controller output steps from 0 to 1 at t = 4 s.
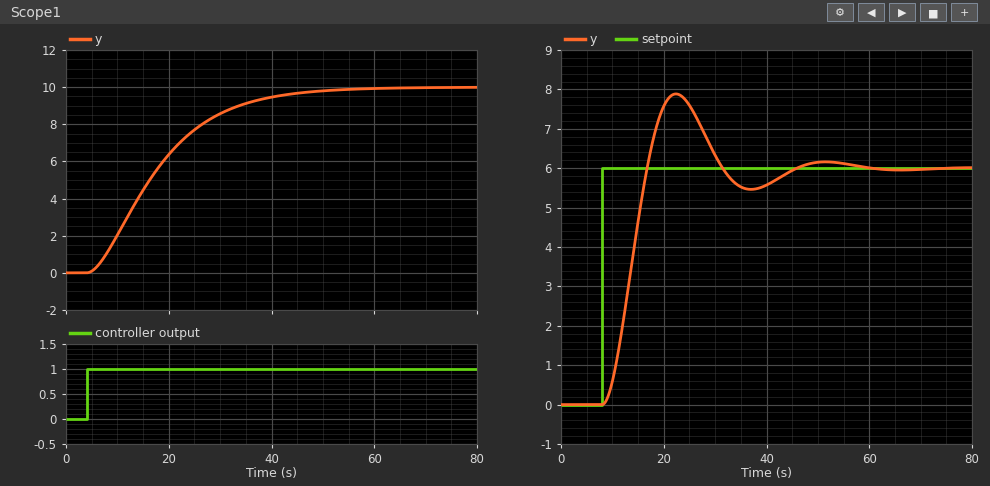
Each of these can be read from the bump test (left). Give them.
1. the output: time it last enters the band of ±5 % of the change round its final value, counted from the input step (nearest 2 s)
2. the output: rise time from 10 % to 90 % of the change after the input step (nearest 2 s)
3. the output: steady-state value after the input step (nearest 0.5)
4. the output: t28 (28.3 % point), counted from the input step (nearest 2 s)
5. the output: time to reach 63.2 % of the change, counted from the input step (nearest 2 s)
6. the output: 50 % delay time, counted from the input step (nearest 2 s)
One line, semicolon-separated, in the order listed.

36 s; 26 s; 10.0; 8 s; 16 s; 12 s
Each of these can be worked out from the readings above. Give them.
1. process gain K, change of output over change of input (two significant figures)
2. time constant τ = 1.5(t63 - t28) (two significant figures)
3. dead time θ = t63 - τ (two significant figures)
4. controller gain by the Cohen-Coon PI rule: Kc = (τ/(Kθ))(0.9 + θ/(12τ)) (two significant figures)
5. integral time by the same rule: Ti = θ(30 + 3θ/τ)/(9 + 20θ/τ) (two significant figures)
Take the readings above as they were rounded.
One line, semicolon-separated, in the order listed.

10; 12 s; 4.0 s; 0.28; 7.9 s
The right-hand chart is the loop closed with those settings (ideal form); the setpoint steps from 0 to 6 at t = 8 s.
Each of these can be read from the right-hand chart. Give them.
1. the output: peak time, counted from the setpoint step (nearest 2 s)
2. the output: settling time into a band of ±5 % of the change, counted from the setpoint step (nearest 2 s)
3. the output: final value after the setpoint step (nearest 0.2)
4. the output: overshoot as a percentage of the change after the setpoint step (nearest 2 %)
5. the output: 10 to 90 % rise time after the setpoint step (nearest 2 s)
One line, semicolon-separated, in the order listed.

14 s; 34 s; 6.0; 32 %; 6 s
